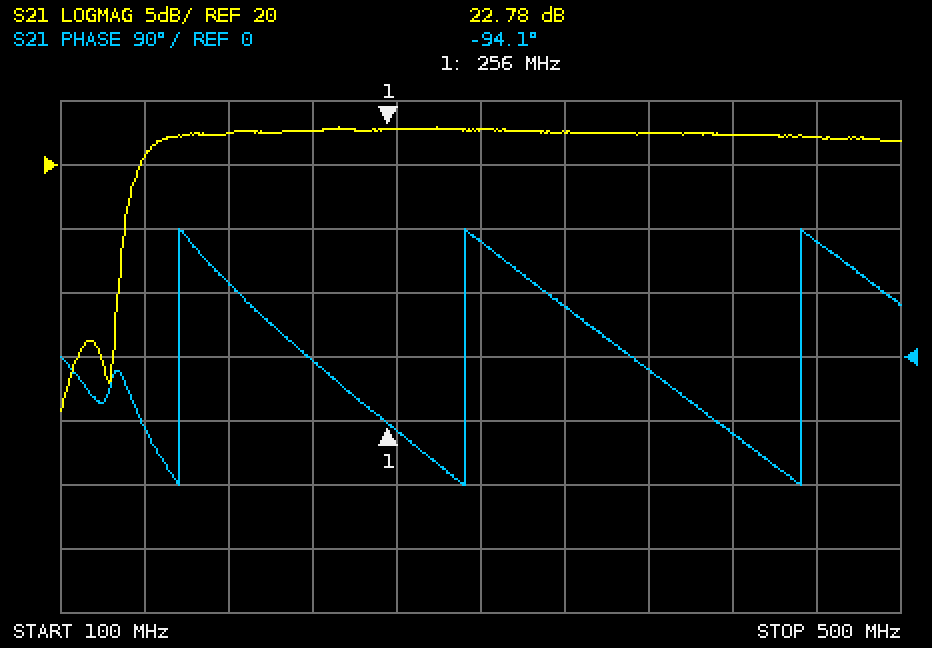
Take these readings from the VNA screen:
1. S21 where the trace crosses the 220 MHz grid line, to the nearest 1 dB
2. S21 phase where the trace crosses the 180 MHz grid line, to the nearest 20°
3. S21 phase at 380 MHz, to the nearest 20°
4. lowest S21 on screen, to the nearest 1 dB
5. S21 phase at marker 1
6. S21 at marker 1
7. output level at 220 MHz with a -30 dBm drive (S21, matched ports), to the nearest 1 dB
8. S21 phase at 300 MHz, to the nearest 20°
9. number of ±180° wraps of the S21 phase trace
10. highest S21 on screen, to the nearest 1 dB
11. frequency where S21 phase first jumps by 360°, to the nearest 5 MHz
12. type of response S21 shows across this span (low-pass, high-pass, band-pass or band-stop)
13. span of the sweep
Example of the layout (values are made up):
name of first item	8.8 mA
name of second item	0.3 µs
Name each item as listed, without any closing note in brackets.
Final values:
S21 where the trace crosses the 220 MHz grid line, to the nearest 1 dB	23 dB
S21 phase where the trace crosses the 180 MHz grid line, to the nearest 20°	100°
S21 phase at 380 MHz, to the nearest 20°	-20°
lowest S21 on screen, to the nearest 1 dB	1 dB
S21 phase at marker 1	-94.1°
S21 at marker 1	22.78 dB
output level at 220 MHz with a -30 dBm drive (S21, matched ports), to the nearest 1 dB	-7 dBm
S21 phase at 300 MHz, to the nearest 20°	160°
number of ±180° wraps of the S21 phase trace	3
highest S21 on screen, to the nearest 1 dB	23 dB
frequency where S21 phase first jumps by 360°, to the nearest 5 MHz	155 MHz
type of response S21 shows across this span	high-pass
span of the sweep	400 MHz
